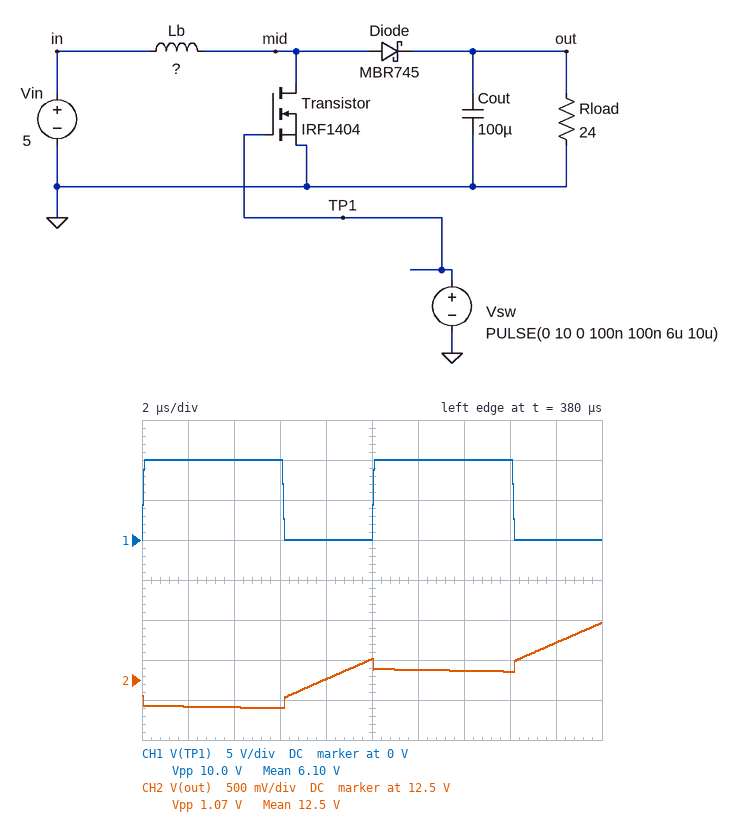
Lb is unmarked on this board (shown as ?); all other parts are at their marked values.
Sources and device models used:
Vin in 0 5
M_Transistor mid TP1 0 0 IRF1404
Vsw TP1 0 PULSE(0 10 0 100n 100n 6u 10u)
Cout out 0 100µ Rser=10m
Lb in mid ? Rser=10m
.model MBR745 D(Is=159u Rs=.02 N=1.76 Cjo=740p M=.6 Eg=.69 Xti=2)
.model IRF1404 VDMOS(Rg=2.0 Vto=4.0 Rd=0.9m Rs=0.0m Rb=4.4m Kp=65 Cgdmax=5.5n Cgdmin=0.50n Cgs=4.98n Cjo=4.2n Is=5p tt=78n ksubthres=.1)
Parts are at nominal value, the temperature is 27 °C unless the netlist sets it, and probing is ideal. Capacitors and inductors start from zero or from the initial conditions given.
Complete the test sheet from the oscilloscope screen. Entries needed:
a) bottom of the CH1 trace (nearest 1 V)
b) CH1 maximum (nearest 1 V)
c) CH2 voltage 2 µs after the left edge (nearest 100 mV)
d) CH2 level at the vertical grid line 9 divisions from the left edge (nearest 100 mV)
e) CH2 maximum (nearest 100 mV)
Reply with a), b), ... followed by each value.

a) 0 V
b) 10 V
c) 12.2 V
d) 13.0 V
e) 13.2 V
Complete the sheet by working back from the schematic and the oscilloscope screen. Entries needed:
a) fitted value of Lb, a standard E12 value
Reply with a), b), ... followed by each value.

a) 82 µH
